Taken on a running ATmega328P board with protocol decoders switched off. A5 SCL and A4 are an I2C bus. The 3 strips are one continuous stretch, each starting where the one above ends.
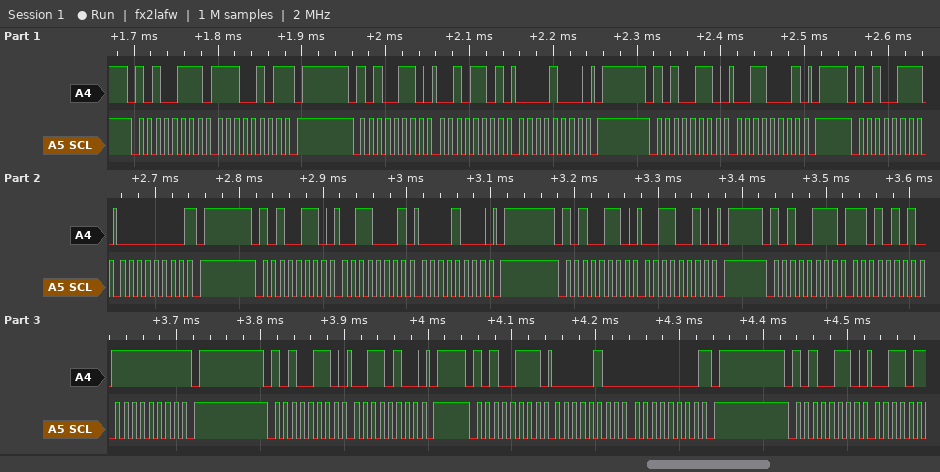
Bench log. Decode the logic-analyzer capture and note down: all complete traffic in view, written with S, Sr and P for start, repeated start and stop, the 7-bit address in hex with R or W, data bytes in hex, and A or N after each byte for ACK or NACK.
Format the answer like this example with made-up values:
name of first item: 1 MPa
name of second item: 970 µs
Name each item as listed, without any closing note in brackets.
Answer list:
all complete traffic in view, written with S, Sr and P for start, repeated start and stop, the 7-bit address in hex with R or W, data bytes in hex, and A or N after each byte for ACK or NACK: S 53R A E5 N P S 53W A 2D A 08 A P S 53W A 31 A P S 53R A 00 N P S 53W A 31 A 08 A P S 53W A 32 A P S 53R A D5 A FF N P S 53W A 34 A P S 53R A 04 A 00 N P S 53W A
